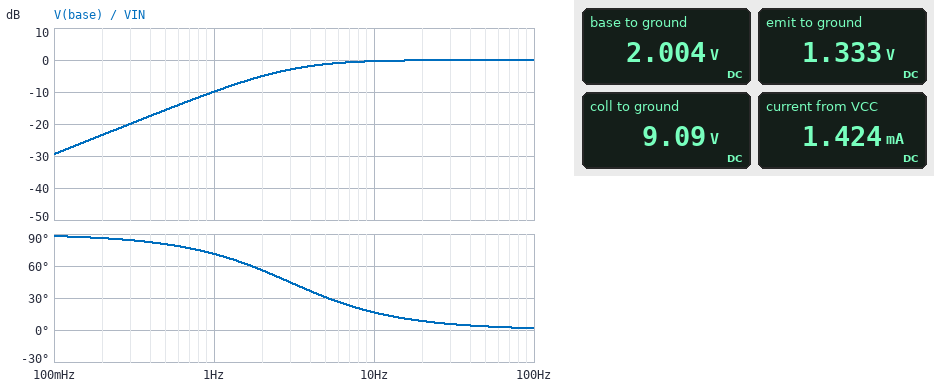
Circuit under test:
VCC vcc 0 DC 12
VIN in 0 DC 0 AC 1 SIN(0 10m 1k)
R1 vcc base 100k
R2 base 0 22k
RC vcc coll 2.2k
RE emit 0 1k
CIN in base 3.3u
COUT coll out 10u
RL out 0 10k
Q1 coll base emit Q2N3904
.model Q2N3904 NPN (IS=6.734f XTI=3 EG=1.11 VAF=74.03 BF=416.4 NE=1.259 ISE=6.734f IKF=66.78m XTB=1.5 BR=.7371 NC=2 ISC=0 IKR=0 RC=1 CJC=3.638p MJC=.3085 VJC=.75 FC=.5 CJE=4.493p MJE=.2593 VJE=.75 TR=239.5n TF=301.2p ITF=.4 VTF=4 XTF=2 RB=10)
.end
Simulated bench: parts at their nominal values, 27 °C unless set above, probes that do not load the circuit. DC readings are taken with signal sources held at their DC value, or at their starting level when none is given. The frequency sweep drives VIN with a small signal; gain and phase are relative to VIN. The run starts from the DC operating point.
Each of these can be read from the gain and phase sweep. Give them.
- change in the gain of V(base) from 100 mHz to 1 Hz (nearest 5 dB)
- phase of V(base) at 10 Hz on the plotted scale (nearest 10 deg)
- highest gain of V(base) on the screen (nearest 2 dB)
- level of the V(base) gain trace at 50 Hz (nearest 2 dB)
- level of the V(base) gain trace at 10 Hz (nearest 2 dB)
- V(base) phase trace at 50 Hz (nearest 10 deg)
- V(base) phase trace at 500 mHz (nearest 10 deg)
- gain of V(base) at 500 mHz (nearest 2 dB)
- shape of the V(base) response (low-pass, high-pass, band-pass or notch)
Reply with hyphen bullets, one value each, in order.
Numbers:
- 20 dB
- 20 deg
- 0 dB
- 0 dB
- 0 dB
- 0 deg
- 80 deg
- -16 dB
- high-pass
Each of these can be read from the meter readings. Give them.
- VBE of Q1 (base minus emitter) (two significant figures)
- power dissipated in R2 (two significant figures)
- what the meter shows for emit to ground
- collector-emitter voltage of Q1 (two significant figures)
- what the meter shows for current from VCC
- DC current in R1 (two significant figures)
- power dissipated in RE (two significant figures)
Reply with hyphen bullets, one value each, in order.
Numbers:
- 670 mV
- 180 µW
- 1.333 V
- 7.8 V
- 1.424 mA
- 100 µA
- 1.8 mW
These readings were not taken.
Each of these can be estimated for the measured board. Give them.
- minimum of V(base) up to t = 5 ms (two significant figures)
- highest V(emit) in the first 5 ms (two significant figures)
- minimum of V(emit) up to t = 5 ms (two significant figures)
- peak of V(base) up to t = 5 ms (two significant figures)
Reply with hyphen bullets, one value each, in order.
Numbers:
- 2.0 V
- 1.3 V
- 1.3 V
- 2.0 V
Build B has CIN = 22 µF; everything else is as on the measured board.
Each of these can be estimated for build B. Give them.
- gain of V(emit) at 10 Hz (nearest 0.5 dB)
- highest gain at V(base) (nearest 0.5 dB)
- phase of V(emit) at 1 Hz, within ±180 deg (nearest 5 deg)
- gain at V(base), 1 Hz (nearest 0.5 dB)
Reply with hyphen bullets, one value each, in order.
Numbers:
- 0 dB
- 0 dB
- 25 deg
- -1.0 dB
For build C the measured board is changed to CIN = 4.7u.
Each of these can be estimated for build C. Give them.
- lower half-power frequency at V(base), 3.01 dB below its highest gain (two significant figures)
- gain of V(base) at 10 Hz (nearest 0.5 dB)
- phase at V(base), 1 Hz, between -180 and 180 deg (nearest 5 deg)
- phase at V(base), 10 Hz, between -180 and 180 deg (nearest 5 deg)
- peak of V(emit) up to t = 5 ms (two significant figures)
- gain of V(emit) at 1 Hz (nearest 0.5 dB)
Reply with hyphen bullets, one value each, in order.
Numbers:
- 2.1 Hz
- 0 dB
- 65 deg
- 10 deg
- 1.3 V
- -7.5 dB
